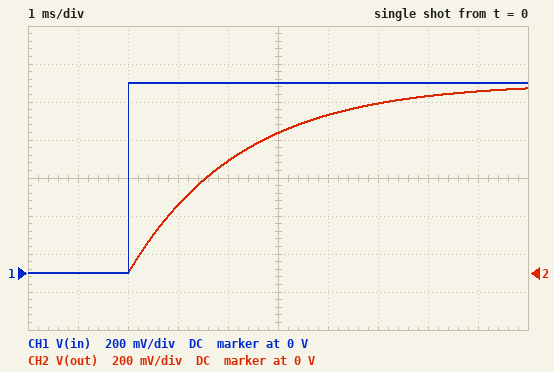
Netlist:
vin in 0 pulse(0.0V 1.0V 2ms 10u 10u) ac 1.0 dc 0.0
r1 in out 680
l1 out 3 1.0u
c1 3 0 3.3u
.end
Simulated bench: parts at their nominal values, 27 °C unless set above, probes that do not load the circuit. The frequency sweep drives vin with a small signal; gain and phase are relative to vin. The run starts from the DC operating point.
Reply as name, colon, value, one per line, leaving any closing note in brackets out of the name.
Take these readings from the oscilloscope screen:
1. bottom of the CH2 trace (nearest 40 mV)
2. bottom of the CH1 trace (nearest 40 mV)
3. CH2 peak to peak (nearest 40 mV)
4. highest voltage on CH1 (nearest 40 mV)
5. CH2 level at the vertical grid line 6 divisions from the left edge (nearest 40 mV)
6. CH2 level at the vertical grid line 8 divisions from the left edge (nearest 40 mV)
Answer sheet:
bottom of the CH2 trace: 0 V
bottom of the CH1 trace: 0 V
CH2 peak to peak: 960 mV
highest voltage on CH1: 1.00 V
CH2 level at the vertical grid line 6 divisions from the left edge: 840 mV
CH2 level at the vertical grid line 8 divisions from the left edge: 920 mV
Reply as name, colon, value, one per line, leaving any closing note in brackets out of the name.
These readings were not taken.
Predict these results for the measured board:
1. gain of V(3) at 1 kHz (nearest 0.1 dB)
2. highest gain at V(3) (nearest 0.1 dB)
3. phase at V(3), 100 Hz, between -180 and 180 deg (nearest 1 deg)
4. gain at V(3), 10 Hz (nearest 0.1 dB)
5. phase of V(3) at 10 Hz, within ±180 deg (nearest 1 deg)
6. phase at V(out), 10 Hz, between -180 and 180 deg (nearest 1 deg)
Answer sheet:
gain of V(3) at 1 kHz: -23.0 dB
highest gain at V(3): 0 dB
phase at V(3), 100 Hz, between -180 and 180 deg: -55 deg
gain at V(3), 10 Hz: -0.1 dB
phase of V(3) at 10 Hz, within ±180 deg: -8 deg
phase at V(out), 10 Hz, between -180 and 180 deg: -8 deg
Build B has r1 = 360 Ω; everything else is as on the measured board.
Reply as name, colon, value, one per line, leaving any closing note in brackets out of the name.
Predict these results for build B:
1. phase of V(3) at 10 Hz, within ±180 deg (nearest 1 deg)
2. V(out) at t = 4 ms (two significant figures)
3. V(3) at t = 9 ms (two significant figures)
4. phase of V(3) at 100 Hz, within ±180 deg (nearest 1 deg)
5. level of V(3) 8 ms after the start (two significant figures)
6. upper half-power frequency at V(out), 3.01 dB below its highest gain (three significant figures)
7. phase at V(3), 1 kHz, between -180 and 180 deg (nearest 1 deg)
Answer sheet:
phase of V(3) at 10 Hz, within ±180 deg: -4 deg
V(out) at t = 4 ms: 810 mV
V(3) at t = 9 ms: 1.0 V
phase of V(3) at 100 Hz, within ±180 deg: -37 deg
level of V(3) 8 ms after the start: 990 mV
upper half-power frequency at V(out), 3.01 dB below its highest gain: 134 Hz
phase at V(3), 1 kHz, between -180 and 180 deg: -82 deg
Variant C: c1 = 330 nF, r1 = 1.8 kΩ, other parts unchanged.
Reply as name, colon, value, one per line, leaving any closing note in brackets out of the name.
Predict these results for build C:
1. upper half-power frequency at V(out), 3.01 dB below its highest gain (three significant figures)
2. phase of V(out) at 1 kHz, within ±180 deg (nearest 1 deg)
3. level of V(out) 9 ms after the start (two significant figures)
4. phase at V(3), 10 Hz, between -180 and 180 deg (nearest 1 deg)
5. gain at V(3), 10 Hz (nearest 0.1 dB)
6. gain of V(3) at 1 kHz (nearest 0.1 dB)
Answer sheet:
upper half-power frequency at V(out), 3.01 dB below its highest gain: 268 Hz
phase of V(out) at 1 kHz, within ±180 deg: -75 deg
level of V(out) 9 ms after the start: 1.0 V
phase at V(3), 10 Hz, between -180 and 180 deg: -2 deg
gain at V(3), 10 Hz: 0 dB
gain of V(3) at 1 kHz: -11.7 dB
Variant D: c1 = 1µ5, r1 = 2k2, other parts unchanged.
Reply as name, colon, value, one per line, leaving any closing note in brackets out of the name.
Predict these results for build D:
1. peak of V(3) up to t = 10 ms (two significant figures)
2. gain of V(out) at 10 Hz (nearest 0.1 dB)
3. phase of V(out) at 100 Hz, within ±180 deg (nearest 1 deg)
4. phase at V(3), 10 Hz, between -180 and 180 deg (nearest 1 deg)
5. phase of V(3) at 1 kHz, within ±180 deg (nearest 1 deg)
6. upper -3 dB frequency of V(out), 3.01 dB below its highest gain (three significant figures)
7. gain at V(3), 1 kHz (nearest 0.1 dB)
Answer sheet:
peak of V(3) up to t = 10 ms: 910 mV
gain of V(out) at 10 Hz: -0.2 dB
phase of V(out) at 100 Hz, within ±180 deg: -64 deg
phase at V(3), 10 Hz, between -180 and 180 deg: -12 deg
phase of V(3) at 1 kHz, within ±180 deg: -87 deg
upper -3 dB frequency of V(out), 3.01 dB below its highest gain: 48.2 Hz
gain at V(3), 1 kHz: -26.3 dB
